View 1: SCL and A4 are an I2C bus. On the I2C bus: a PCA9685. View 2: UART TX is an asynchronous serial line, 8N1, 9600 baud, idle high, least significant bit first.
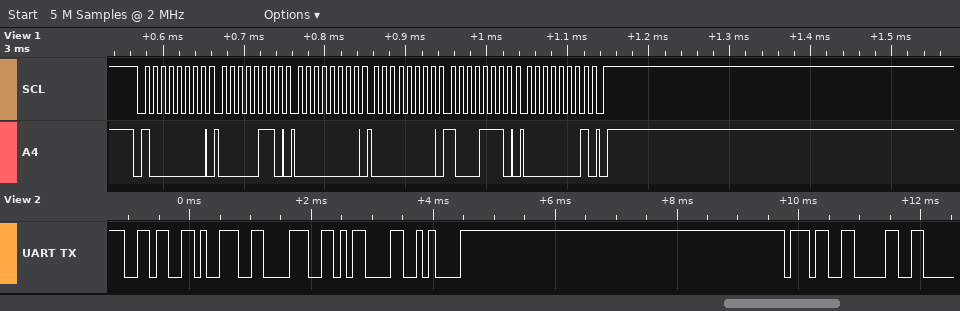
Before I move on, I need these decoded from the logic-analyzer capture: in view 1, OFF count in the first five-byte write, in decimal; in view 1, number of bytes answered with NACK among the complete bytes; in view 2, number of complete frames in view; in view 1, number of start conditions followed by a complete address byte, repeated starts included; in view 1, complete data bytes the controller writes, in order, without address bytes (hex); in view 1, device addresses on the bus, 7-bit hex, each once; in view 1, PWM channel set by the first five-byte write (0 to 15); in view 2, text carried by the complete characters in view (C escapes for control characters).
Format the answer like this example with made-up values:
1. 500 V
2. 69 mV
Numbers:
1. 398
2. 0
3. 7
4. 1
5. 06 00 00 8E 01
6. 0x40
7. 0
8. "698\r\n70"
